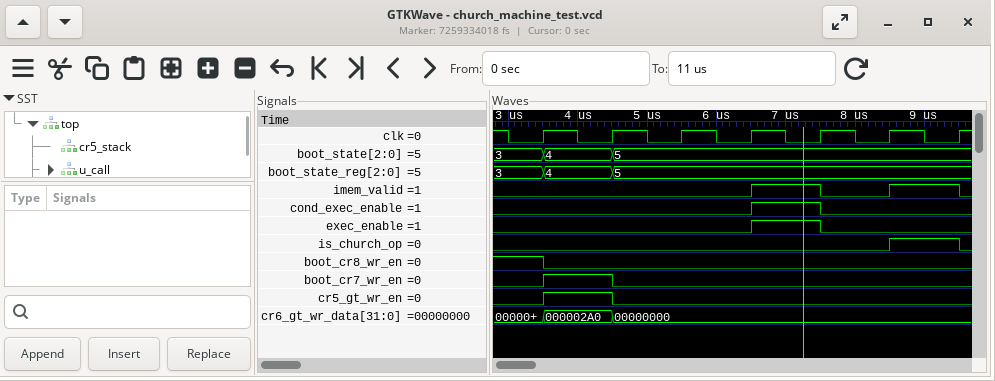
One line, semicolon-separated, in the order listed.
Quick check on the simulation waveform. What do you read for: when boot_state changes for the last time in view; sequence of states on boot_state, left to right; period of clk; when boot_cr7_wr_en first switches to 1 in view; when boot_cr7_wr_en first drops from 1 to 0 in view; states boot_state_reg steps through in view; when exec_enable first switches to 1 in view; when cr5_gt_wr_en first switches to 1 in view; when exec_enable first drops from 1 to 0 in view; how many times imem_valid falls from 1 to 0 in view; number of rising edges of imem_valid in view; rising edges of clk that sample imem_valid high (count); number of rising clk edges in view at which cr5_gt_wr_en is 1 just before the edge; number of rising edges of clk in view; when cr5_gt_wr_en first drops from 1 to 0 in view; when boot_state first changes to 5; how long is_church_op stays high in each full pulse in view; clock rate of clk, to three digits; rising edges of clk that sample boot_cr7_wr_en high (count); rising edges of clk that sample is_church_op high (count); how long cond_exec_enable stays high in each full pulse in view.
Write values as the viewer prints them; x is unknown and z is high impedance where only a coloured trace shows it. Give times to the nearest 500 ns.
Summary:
4500 ns; 3, 4, 5; 1000 ns; 3500 ns; 4500 ns; 3, 4, 5; 6500 ns; 3500 ns; 7500 ns; 2; 2; 2; 1; 7; 4500 ns; 4500 ns; 1000 ns; 1.00 MHz; 1; 1; 1000 ns
